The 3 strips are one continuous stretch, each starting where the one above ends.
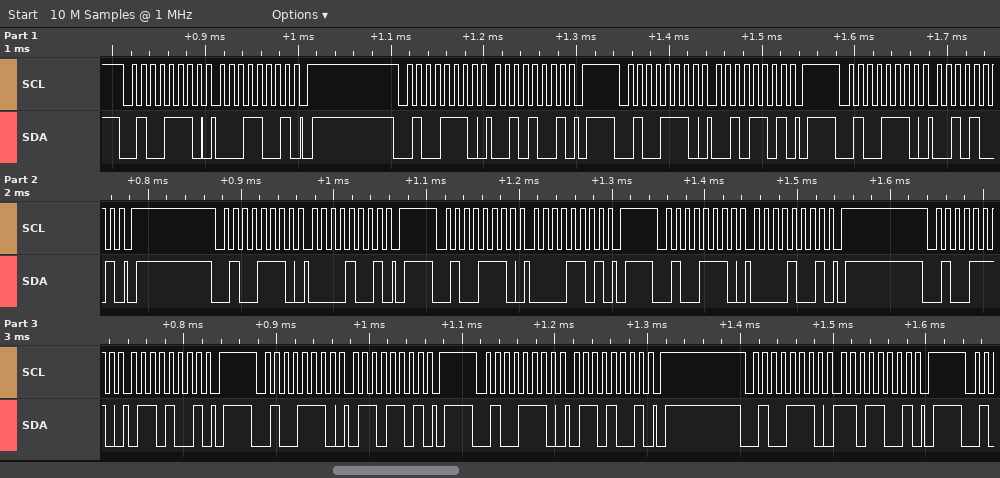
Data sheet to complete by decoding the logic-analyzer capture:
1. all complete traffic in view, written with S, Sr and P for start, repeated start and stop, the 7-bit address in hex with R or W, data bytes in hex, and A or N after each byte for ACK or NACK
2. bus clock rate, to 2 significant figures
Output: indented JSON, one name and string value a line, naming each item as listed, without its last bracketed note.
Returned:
{
  "all complete traffic in view, written with S, Sr and P for start, repeated start and stop, the 7-bit address in hex with R or W, data bytes in hex, and A or N after each byte for ACK or NACK": "S 27W A 19 A P S 27W A 29 A P S 27W A 2D A P S 27W A 29 A P S 27W A 09 A P S 27W A 0D A P S 27W A 09 A P S 27W A 69 A P S 27W A 6D A P S 27W A 69 A P S 27W A D9 A P",
  "bus clock rate, to 2 significant figures": "100 kHz"
}
